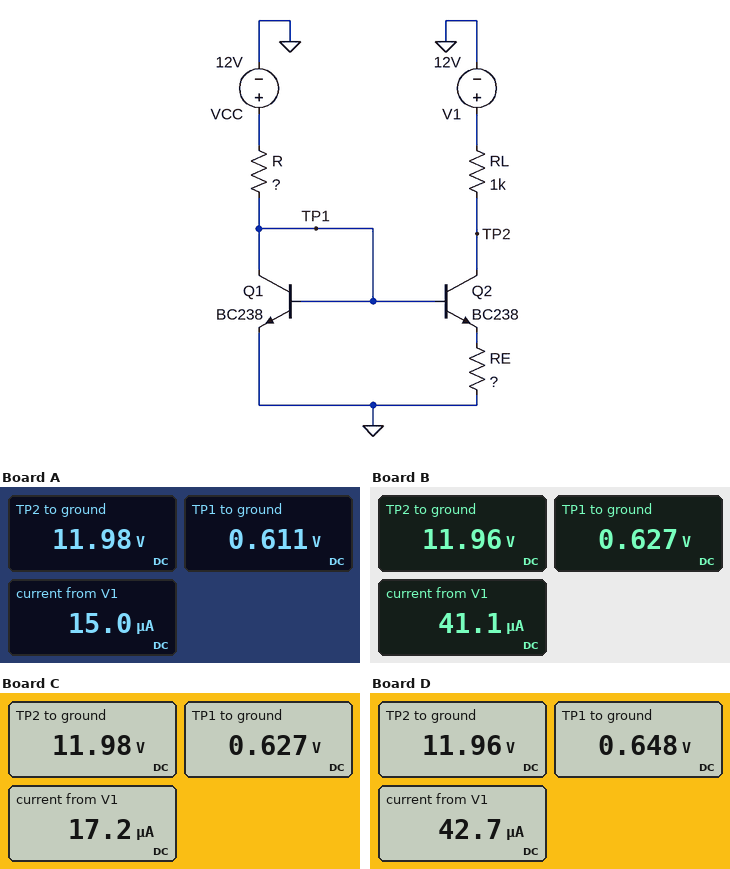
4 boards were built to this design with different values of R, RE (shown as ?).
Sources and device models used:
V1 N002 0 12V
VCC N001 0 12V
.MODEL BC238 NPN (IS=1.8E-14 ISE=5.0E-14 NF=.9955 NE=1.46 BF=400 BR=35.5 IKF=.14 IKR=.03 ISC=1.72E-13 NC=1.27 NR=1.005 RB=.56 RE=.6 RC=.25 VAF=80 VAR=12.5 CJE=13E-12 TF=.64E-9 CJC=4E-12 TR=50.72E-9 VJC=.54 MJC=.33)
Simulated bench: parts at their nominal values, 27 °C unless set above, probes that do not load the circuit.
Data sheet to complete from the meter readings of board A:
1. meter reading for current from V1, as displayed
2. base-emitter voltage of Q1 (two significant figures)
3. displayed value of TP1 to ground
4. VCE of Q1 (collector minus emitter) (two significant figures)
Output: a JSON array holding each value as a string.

["15.0 µA", "610 mV", "0.611 V", "610 mV"]
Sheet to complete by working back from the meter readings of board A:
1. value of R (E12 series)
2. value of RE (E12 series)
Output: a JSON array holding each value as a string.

["33 kΩ", "5.6 kΩ"]
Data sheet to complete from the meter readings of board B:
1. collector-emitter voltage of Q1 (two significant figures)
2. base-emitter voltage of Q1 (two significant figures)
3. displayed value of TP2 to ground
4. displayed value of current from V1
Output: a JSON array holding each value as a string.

["630 mV", "630 mV", "11.96 V", "41.1 µA"]
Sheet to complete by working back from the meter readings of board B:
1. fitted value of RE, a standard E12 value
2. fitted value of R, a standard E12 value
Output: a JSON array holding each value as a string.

["1.8 kΩ", "18 kΩ"]
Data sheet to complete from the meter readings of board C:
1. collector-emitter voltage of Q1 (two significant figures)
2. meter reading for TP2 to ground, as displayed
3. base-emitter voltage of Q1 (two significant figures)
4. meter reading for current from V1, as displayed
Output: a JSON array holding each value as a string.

["630 mV", "11.98 V", "630 mV", "17.2 µA"]
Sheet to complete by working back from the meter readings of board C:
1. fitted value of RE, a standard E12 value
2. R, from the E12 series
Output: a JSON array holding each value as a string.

["5.6 kΩ", "18 kΩ"]
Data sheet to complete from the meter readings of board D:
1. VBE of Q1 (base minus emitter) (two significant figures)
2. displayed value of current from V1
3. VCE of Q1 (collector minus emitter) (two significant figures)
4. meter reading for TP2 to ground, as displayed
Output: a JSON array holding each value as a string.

["650 mV", "42.7 µA", "650 mV", "11.96 V"]
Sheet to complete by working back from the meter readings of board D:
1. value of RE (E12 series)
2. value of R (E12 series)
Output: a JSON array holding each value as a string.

["2.2 kΩ", "8.2 kΩ"]
